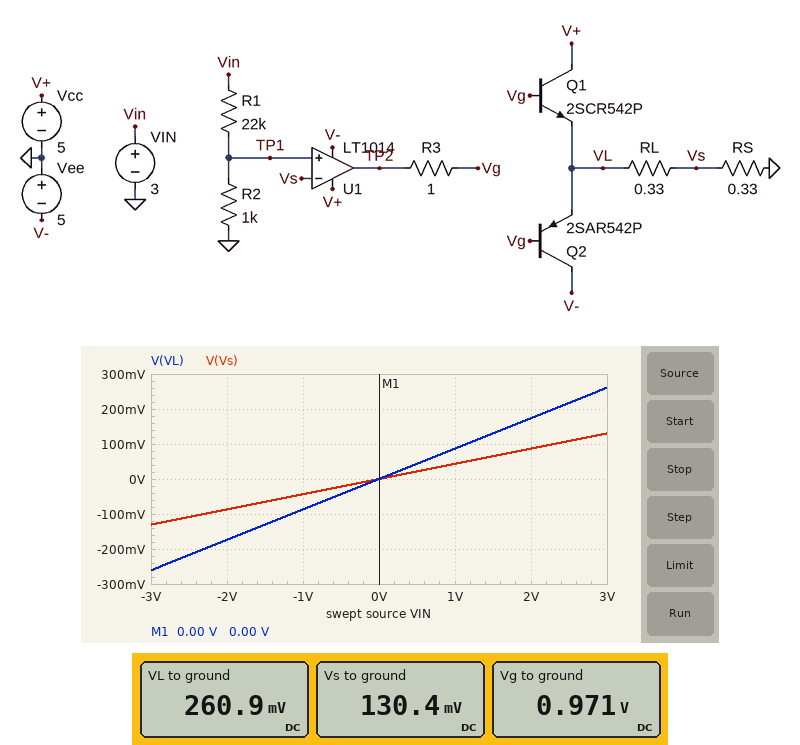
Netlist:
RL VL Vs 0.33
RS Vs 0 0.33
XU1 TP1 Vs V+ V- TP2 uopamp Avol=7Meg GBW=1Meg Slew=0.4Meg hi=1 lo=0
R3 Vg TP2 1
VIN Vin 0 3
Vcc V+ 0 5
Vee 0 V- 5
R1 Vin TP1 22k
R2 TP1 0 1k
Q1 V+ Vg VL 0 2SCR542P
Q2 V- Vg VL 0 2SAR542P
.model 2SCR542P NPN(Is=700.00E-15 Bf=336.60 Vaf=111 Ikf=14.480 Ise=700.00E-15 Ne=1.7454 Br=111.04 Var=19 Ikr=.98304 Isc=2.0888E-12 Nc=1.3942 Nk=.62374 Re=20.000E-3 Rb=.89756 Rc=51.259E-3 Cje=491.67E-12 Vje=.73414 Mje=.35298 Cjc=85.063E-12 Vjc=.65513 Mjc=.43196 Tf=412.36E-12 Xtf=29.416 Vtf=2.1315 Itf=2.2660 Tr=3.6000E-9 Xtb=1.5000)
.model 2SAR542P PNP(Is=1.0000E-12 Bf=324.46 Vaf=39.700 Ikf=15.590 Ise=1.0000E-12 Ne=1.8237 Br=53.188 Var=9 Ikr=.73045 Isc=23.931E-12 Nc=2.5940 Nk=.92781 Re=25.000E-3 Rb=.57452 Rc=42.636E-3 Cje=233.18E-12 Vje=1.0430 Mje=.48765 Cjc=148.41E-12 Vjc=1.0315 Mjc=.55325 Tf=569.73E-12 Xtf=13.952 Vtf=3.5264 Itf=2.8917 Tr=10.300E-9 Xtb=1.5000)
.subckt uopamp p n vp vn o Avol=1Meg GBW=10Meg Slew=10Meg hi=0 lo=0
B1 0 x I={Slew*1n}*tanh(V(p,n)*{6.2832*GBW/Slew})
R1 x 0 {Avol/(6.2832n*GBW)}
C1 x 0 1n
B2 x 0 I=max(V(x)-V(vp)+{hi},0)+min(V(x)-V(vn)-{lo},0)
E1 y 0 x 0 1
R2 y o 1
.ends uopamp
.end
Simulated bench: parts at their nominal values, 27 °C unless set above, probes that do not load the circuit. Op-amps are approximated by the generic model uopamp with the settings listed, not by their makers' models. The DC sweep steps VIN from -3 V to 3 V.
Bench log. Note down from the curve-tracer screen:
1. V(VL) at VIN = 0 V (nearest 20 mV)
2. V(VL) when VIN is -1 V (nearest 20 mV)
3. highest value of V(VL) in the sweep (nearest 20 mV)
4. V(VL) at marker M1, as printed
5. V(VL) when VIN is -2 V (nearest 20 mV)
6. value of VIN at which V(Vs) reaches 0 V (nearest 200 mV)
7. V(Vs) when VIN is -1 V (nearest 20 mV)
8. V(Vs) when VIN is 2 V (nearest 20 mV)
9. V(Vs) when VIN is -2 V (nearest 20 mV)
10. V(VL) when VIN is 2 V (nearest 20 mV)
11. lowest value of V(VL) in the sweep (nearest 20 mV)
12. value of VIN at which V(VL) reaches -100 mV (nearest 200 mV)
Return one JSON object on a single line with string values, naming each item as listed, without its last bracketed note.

{"V(VL) at VIN = 0 V": "0 V", "V(VL) when VIN is -1 V": "-80 mV", "highest value of V(VL) in the sweep": "260 mV", "V(VL) at marker M1, as printed": "0.00 V", "V(VL) when VIN is -2 V": "-180 mV", "value of VIN at which V(Vs) reaches 0 V": "0 V", "V(Vs) when VIN is -1 V": "-40 mV", "V(Vs) when VIN is 2 V": "80 mV", "V(Vs) when VIN is -2 V": "-80 mV", "V(VL) when VIN is 2 V": "180 mV", "lowest value of V(VL) in the sweep": "-260 mV", "value of VIN at which V(VL) reaches -100 mV": "-1.2 V"}
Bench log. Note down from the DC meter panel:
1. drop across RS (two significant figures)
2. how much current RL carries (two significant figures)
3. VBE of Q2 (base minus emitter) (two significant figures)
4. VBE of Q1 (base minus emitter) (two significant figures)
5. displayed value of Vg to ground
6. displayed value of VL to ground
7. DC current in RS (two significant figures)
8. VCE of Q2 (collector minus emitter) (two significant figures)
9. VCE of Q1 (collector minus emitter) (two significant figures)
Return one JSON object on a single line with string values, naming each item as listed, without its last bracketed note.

{"drop across RS": "130 mV", "how much current RL carries": "400 mA", "VBE of Q2 (base minus emitter)": "710 mV", "VBE of Q1 (base minus emitter)": "710 mV", "displayed value of Vg to ground": "0.971 V", "displayed value of VL to ground": "260.9 mV", "DC current in RS": "400 mA", "VCE of Q2 (collector minus emitter)": "-5.3 V", "VCE of Q1 (collector minus emitter)": "4.7 V"}
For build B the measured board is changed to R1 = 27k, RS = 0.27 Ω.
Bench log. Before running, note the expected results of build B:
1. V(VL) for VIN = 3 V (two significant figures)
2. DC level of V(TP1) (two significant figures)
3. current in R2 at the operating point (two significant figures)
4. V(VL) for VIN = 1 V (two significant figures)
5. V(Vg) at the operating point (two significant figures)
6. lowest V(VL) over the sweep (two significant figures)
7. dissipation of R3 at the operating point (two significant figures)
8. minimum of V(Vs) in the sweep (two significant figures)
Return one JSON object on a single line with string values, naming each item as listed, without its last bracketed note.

{"V(VL) for VIN = 3 V": "240 mV", "DC level of V(TP1)": "110 mV", "current in R2 at the operating point": "110 µA", "V(VL) for VIN = 1 V": "79 mV", "V(Vg) at the operating point": "950 mV", "lowest V(VL) over the sweep": "-240 mV", "dissipation of R3 at the operating point": "1.5 µW", "minimum of V(Vs) in the sweep": "-110 mV"}
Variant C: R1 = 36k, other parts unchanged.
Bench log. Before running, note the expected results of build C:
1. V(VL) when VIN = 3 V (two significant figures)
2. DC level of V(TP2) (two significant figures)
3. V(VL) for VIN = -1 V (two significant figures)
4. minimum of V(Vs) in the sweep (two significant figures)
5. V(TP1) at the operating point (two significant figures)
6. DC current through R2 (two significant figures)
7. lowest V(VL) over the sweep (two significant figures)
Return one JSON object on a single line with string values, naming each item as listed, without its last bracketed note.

{"V(VL) when VIN = 3 V": "160 mV", "DC level of V(TP2)": "860 mV", "V(VL) for VIN = -1 V": "-54 mV", "minimum of V(Vs) in the sweep": "-81 mV", "V(TP1) at the operating point": "81 mV", "DC current through R2": "81 µA", "lowest V(VL) over the sweep": "-160 mV"}
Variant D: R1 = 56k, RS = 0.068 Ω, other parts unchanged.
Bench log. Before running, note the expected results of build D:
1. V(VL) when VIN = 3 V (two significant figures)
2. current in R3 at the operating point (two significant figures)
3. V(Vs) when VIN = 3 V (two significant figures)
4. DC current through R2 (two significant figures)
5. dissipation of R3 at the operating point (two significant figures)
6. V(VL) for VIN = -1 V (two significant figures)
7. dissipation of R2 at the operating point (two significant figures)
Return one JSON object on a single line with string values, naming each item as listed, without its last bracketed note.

{"V(VL) when VIN = 3 V": "310 mV", "current in R3 at the operating point": "2.5 mA", "V(Vs) when VIN = 3 V": "53 mV", "DC current through R2": "53 µA", "dissipation of R3 at the operating point": "6.1 µW", "V(VL) for VIN = -1 V": "-100 mV", "dissipation of R2 at the operating point": "2.8 µW"}
